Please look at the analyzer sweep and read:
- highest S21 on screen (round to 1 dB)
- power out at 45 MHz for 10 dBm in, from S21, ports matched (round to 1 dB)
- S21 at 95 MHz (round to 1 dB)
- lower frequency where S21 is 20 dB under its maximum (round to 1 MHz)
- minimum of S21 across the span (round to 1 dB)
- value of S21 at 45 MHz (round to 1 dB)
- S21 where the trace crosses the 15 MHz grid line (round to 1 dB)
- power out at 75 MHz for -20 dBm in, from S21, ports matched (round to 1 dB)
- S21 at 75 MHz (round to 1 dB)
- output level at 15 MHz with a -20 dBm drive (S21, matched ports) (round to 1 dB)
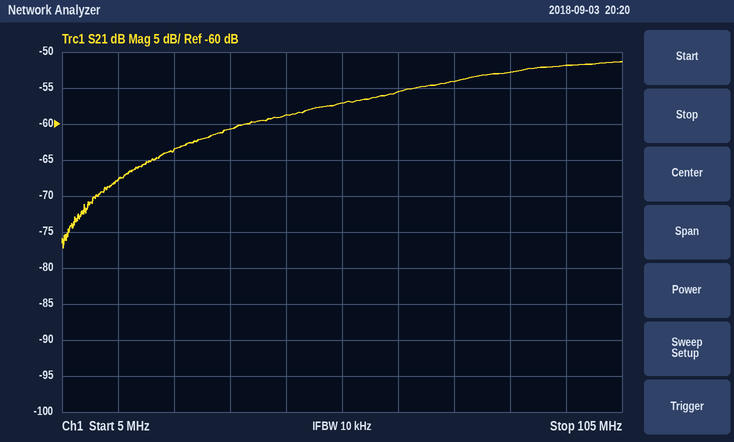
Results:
-51 dB
-49 dBm
-52 dB
10 MHz
-77 dB
-59 dB
-68 dB
-74 dBm
-54 dB
-88 dBm
